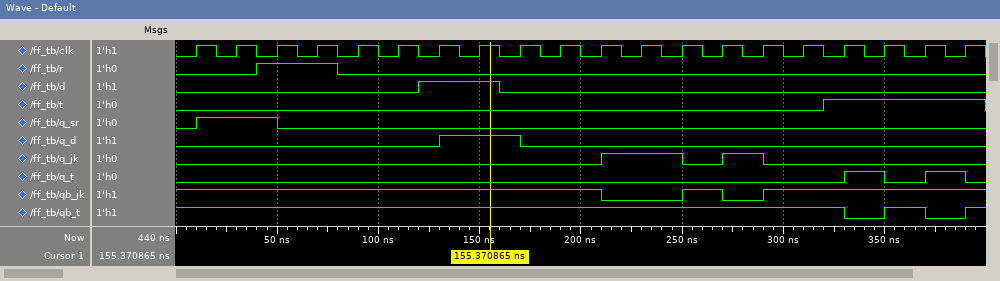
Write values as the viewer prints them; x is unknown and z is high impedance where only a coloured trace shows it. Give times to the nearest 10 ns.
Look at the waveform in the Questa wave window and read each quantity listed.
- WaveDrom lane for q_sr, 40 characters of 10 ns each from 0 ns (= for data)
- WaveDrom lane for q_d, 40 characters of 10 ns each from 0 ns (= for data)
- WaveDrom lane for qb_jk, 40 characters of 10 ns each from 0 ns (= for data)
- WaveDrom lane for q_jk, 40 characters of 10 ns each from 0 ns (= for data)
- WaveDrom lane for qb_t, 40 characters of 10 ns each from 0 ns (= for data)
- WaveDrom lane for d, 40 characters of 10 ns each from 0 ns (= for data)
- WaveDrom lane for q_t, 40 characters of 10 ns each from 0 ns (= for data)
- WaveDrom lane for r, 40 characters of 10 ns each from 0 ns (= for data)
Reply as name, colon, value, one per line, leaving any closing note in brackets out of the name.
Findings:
WaveDrom lane for q_sr, 40 characters of 10 ns each from 0 ns: {name: 'q_sr', wave: '01...0..................................'}
WaveDrom lane for q_d, 40 characters of 10 ns each from 0 ns: {name: 'q_d', wave: '0............1...0......................'}
WaveDrom lane for qb_jk, 40 characters of 10 ns each from 0 ns: {name: 'qb_jk', wave: '1....................0...1.0.1..........'}
WaveDrom lane for q_jk, 40 characters of 10 ns each from 0 ns: {name: 'q_jk', wave: '0....................1...0.1.0..........'}
WaveDrom lane for qb_t, 40 characters of 10 ns each from 0 ns: {name: 'qb_t', wave: '1................................0.1.0.1'}
WaveDrom lane for d, 40 characters of 10 ns each from 0 ns: {name: 'd', wave: '0...........1...0.......................'}
WaveDrom lane for q_t, 40 characters of 10 ns each from 0 ns: {name: 'q_t', wave: '0................................1.0.1.0'}
WaveDrom lane for r, 40 characters of 10 ns each from 0 ns: {name: 'r', wave: '0...1...0...............................'}
